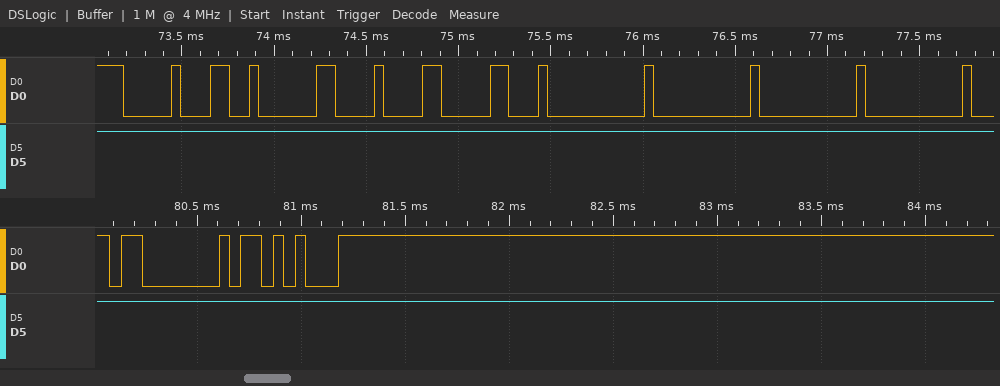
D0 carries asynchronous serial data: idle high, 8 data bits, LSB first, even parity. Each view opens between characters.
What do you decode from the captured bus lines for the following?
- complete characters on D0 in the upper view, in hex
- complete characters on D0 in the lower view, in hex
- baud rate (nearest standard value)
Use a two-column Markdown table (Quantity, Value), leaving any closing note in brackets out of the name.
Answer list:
| Quantity | Value |
|---|---|
| complete characters on D0 in the upper view, in hex | 10, 02, 08, 30, 00, 00, 00, 00 |
| complete characters on D0 in the lower view, in hex | 03, 2B |
| baud rate | 19200 baud |
